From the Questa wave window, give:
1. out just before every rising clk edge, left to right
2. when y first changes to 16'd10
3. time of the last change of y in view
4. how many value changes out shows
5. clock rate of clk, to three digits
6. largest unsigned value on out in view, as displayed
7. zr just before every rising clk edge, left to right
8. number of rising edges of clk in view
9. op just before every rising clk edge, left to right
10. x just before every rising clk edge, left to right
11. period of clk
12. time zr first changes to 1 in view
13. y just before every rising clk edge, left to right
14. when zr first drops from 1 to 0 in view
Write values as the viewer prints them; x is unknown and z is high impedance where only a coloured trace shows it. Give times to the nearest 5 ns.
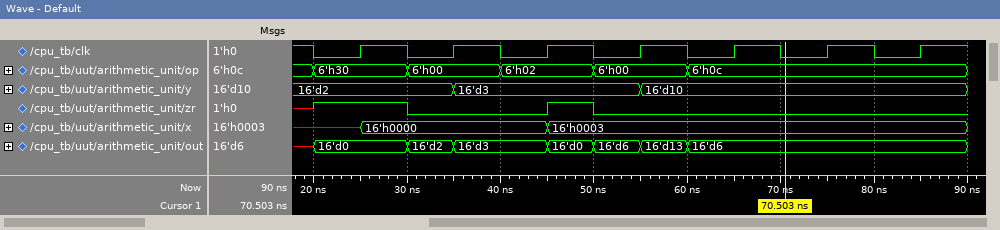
16'd0, 16'd2, 16'd3, 16'd6, 16'd6, 16'd6, 16'd6
55 ns
55 ns
7
100 MHz
16'd13
1 0 0 0 0 0 0
7
6'h30, 6'h00, 6'h02, 6'h00, 6'h0c, 6'h0c, 6'h0c
x, 16'h0000, 16'h0000, 16'h0003, 16'h0003, 16'h0003, 16'h0003
10 ns
20 ns
16'd2, 16'd2, 16'd3, 16'd3, 16'd10, 16'd10, 16'd10
30 ns
